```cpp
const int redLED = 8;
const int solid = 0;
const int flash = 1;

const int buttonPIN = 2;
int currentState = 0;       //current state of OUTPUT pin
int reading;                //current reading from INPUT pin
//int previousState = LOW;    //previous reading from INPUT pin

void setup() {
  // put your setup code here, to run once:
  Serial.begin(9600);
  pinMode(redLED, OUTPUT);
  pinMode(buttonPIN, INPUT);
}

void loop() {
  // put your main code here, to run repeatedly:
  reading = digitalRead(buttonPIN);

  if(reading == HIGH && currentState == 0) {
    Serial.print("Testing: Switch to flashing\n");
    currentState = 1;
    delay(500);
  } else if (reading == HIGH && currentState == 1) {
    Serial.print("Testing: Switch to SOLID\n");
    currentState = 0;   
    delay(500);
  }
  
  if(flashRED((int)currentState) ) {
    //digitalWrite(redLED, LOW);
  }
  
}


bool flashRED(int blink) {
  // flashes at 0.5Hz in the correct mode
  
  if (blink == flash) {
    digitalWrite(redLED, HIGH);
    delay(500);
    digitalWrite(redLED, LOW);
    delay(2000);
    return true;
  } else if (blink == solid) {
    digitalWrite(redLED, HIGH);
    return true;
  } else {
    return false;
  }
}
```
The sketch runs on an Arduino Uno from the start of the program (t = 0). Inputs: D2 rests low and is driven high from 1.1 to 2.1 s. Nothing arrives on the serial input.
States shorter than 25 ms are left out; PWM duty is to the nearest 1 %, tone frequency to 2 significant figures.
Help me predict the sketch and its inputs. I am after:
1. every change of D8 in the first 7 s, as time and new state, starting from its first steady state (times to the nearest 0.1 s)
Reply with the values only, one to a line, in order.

0 s high; 2.1 s low; 4.1 s high; 4.6 s low; 6.6 s high
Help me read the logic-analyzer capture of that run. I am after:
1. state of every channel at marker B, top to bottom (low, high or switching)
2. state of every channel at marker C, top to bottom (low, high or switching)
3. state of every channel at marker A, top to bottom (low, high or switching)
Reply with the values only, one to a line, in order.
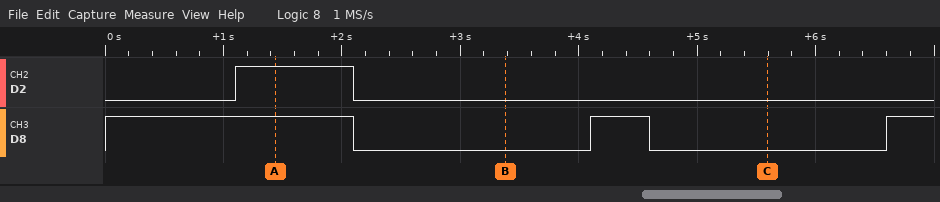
D2 low, D8 low
D2 low, D8 low
D2 high, D8 high
